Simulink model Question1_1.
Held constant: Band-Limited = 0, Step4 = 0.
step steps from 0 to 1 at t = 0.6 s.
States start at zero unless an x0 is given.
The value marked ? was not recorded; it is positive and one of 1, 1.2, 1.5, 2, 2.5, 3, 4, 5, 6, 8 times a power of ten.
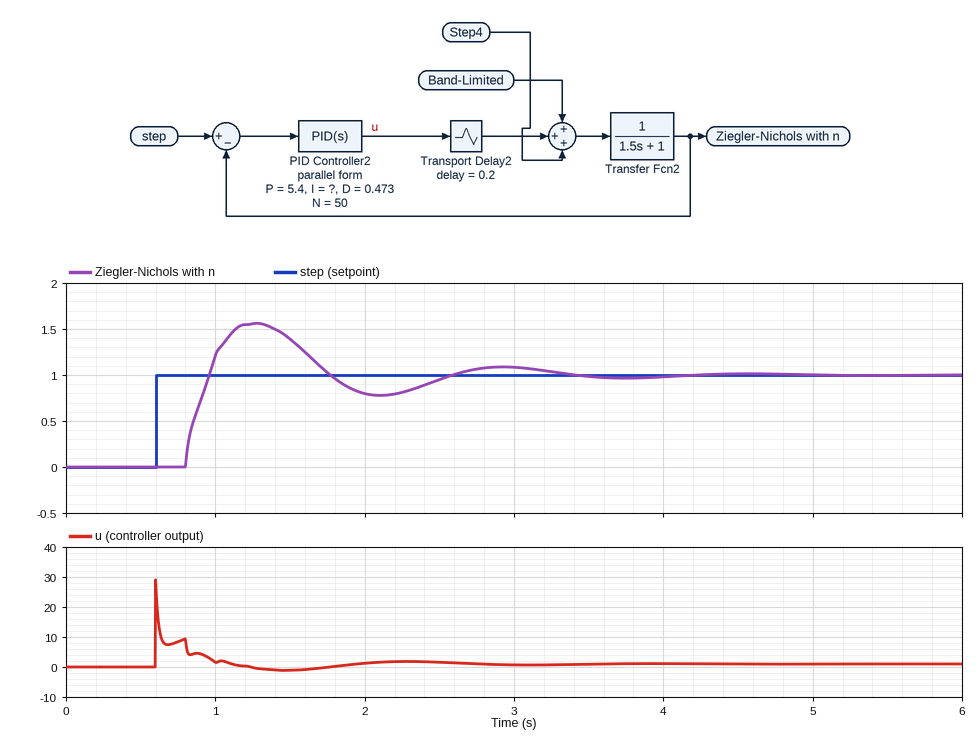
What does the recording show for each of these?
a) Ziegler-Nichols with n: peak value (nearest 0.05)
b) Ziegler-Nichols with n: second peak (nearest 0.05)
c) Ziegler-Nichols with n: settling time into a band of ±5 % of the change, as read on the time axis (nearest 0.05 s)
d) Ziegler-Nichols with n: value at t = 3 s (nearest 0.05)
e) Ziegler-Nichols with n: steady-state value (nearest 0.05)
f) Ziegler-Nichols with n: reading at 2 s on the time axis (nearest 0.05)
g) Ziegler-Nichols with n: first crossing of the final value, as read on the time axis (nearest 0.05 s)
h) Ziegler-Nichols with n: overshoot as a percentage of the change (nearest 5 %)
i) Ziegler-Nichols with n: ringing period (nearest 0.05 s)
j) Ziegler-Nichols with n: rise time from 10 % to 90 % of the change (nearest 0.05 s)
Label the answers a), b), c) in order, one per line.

a) 1.55
b) 1.10
c) 3.20 s
d) 1.10
e) 1.00
f) 0.80
g) 0.95 s
h) 55 %
i) 1.65 s
j) 0.15 s
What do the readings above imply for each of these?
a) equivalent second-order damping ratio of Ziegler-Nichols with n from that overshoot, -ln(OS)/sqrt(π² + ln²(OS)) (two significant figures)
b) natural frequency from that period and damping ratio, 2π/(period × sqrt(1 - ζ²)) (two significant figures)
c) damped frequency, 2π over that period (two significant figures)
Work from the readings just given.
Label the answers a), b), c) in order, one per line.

a) 0.19
b) 3.9 rad/s
c) 3.8 rad/s
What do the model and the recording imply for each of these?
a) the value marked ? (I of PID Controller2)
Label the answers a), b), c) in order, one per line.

a) 20
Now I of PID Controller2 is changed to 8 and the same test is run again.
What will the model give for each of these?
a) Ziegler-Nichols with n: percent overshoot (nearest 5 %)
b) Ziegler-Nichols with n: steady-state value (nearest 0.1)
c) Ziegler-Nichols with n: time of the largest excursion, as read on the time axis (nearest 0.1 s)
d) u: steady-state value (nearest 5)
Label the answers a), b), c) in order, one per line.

a) 15 %
b) 1.0
c) 1.6 s
d) 0
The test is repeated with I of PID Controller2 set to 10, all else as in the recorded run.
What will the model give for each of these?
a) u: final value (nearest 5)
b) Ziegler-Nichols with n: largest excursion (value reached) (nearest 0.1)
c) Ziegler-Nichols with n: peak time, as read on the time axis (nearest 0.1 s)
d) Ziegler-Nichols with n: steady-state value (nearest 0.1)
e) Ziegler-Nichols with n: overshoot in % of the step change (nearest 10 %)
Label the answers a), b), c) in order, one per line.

a) 0
b) 1.2
c) 1.2 s
d) 1.0
e) 20 %
